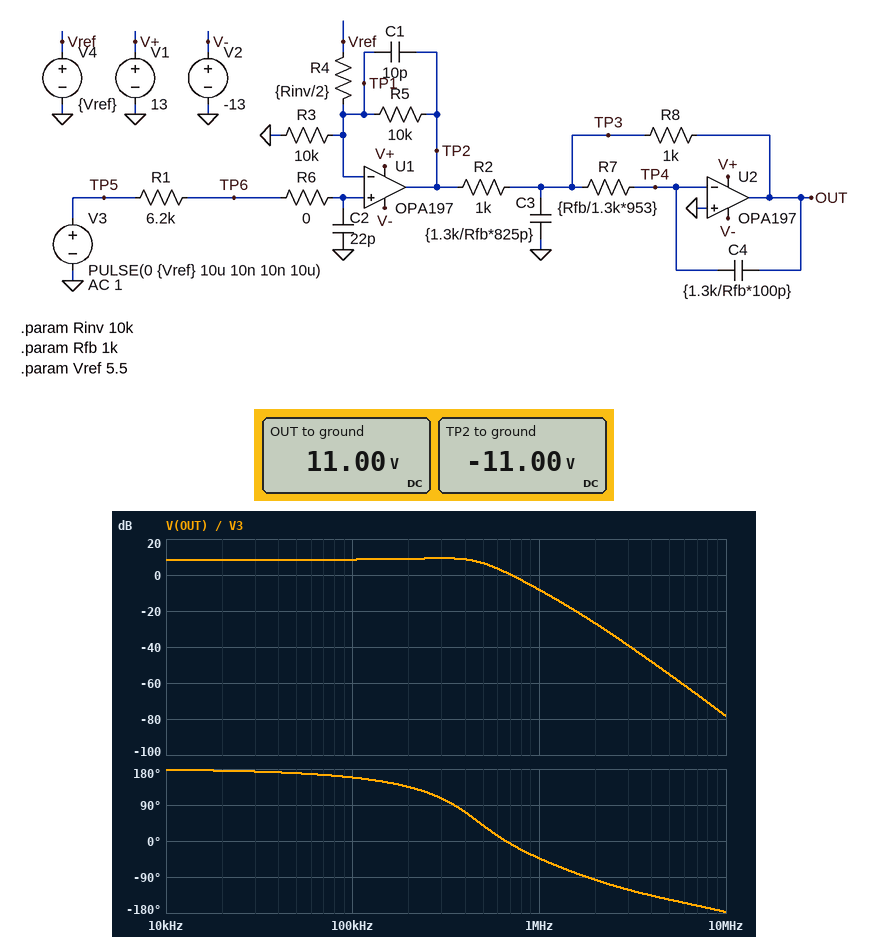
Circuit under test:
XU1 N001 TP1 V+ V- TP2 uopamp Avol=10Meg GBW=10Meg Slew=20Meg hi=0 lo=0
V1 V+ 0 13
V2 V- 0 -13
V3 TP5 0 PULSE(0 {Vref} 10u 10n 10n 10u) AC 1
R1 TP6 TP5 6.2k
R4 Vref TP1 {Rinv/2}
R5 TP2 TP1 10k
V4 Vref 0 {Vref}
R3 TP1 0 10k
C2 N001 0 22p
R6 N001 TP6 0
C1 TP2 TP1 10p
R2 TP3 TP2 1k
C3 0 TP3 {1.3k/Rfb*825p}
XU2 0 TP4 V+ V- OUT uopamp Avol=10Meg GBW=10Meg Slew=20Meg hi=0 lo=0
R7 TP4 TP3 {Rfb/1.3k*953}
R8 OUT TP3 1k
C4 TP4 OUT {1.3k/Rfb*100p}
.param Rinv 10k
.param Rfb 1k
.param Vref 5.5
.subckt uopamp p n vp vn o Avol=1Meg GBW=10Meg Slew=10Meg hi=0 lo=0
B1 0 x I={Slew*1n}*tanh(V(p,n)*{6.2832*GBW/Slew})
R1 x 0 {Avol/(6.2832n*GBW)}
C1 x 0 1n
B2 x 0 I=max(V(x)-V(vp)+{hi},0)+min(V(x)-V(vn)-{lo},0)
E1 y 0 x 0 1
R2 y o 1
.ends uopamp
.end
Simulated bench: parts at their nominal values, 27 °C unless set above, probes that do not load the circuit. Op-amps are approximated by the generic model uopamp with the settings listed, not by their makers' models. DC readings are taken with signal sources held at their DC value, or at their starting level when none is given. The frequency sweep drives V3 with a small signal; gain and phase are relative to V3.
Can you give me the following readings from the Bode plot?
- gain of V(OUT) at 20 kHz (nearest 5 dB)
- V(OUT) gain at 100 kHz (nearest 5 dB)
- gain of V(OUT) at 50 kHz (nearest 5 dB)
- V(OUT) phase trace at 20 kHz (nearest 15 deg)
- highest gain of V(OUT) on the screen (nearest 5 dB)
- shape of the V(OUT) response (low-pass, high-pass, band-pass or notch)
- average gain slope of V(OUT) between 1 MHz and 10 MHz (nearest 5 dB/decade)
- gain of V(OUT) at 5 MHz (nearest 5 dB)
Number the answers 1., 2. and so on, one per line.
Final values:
1. 10 dB
2. 10 dB
3. 10 dB
4. 180 deg
5. 10 dB
6. low-pass
7. -70 dB/decade
8. -55 dB
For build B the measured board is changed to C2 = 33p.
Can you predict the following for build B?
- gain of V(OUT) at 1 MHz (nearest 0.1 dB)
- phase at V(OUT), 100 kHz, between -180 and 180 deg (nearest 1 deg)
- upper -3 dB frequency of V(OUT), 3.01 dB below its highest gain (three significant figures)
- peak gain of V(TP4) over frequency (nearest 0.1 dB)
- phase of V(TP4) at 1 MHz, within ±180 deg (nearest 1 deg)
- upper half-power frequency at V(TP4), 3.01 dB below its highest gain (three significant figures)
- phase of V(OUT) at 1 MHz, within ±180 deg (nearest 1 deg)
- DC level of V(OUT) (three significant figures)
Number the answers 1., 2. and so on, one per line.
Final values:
1. -9.4 dB
2. 157 deg
3. 501 kHz
4. -19.4 dB
5. -144 deg
6. 646 kHz
7. -54 deg
8. 11.0 V
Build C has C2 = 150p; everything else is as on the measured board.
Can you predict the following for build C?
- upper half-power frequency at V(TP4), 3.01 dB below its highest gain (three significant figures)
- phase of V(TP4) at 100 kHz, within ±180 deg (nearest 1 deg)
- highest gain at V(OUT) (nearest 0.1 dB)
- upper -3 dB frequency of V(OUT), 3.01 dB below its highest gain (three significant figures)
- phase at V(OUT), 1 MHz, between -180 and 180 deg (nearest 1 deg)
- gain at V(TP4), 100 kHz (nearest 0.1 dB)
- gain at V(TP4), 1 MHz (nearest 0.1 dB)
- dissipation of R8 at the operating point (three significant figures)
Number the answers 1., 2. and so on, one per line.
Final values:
1. 555 kHz
2. 51 deg
3. 8.4 dB
4. 318 kHz
5. -89 deg
6. -32.0 dB
7. -39.0 dB
8. 121 mW
